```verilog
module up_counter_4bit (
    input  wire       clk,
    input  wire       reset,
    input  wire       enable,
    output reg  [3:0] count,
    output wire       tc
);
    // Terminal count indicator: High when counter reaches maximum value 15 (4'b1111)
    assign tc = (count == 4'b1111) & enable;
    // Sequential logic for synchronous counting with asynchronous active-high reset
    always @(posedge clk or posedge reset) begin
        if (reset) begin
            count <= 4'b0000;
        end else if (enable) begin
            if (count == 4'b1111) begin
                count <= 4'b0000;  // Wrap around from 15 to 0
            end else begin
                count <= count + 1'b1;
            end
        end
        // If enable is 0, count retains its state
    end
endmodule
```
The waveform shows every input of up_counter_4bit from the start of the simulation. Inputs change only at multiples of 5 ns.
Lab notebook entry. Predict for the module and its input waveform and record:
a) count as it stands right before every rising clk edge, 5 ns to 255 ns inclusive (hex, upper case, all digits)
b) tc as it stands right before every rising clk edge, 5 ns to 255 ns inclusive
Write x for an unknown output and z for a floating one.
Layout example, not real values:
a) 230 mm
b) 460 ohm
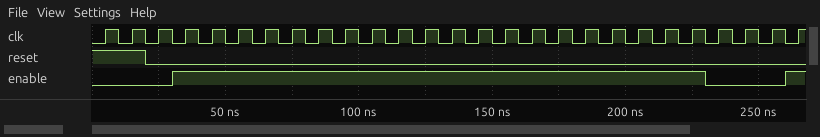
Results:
a) 0, 0, 0, 0, 1, 2, 3, 4, 5, 6, 7, 8, 9, A, B, C, D, E, F, 0, 1, 2, 3, 4, 4, 4
b) 0 0 0 0 0 0 0 0 0 0 0 0 0 0 0 0 0 0 1 0 0 0 0 0 0 0
